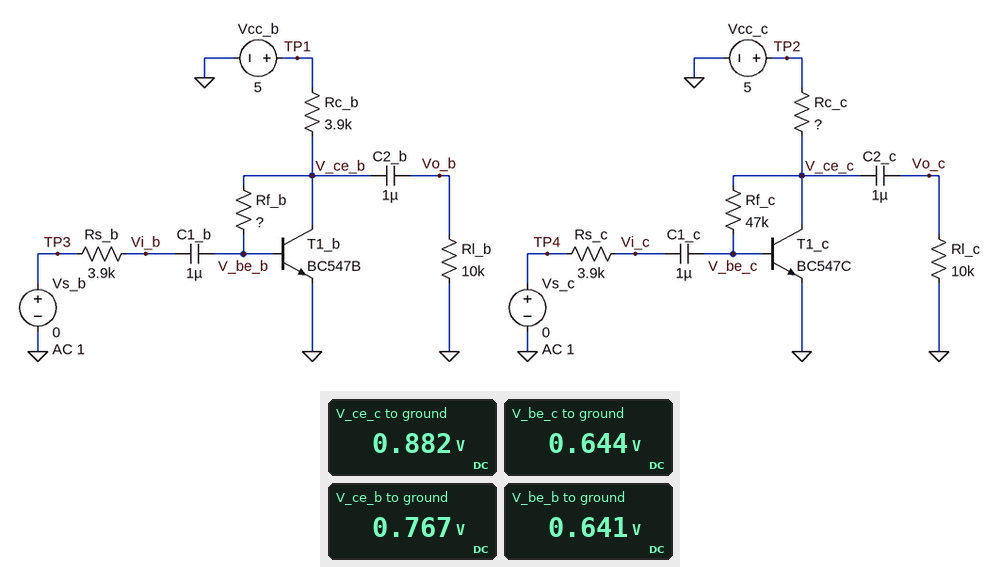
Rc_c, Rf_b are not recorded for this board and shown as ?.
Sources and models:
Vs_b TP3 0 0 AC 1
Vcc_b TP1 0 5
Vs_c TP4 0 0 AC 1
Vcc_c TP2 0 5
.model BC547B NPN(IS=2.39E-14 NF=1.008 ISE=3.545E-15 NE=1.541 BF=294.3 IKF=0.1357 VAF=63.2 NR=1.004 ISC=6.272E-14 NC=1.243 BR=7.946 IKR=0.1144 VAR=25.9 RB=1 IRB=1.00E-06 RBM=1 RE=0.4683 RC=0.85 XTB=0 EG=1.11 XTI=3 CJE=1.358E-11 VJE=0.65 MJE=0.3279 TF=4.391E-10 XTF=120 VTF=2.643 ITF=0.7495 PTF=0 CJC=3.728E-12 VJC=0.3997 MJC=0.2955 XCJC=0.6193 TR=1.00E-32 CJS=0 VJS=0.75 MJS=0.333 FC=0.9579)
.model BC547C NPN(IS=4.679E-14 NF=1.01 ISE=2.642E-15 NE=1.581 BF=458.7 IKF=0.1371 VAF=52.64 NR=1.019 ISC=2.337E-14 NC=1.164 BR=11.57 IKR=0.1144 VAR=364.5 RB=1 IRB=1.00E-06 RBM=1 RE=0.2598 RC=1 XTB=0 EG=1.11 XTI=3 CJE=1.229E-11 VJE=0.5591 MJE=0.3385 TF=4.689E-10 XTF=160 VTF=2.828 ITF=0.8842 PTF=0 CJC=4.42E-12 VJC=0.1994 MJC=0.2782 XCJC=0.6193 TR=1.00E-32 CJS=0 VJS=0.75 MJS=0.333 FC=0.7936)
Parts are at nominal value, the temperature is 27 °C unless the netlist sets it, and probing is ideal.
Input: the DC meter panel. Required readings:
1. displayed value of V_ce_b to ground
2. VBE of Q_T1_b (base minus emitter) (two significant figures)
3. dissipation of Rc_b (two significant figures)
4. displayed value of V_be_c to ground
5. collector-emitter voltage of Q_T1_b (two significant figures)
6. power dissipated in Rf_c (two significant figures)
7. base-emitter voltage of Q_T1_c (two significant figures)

0.767 V
640 mV
4.6 mW
0.644 V
770 mV
1.2 µW
640 mV
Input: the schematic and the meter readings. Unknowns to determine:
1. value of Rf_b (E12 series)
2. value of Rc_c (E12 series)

33 kΩ
1.8 kΩ
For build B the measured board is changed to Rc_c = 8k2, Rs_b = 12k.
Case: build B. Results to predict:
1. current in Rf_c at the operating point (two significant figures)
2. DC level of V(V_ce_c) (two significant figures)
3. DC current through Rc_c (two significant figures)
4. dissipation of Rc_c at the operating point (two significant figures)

1.2 µA
660 mV
530 µA
2.3 mW
